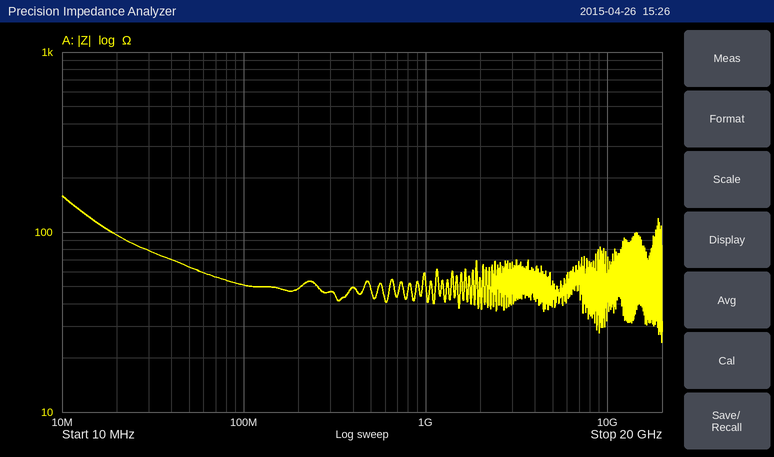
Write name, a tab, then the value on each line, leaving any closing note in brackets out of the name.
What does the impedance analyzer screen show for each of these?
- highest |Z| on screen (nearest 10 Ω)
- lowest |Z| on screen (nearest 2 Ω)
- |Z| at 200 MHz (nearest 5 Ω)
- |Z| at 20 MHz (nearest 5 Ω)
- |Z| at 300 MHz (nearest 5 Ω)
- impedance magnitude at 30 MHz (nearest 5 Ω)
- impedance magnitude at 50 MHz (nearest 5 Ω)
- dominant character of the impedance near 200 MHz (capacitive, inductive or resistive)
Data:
highest |Z| on screen	160 Ω
lowest |Z| on screen	24 Ω
|Z| at 200 MHz	50 Ω
|Z| at 20 MHz	95 Ω
|Z| at 300 MHz	45 Ω
impedance magnitude at 30 MHz	80 Ω
impedance magnitude at 50 MHz	65 Ω
dominant character of the impedance near 200 MHz	resistive
